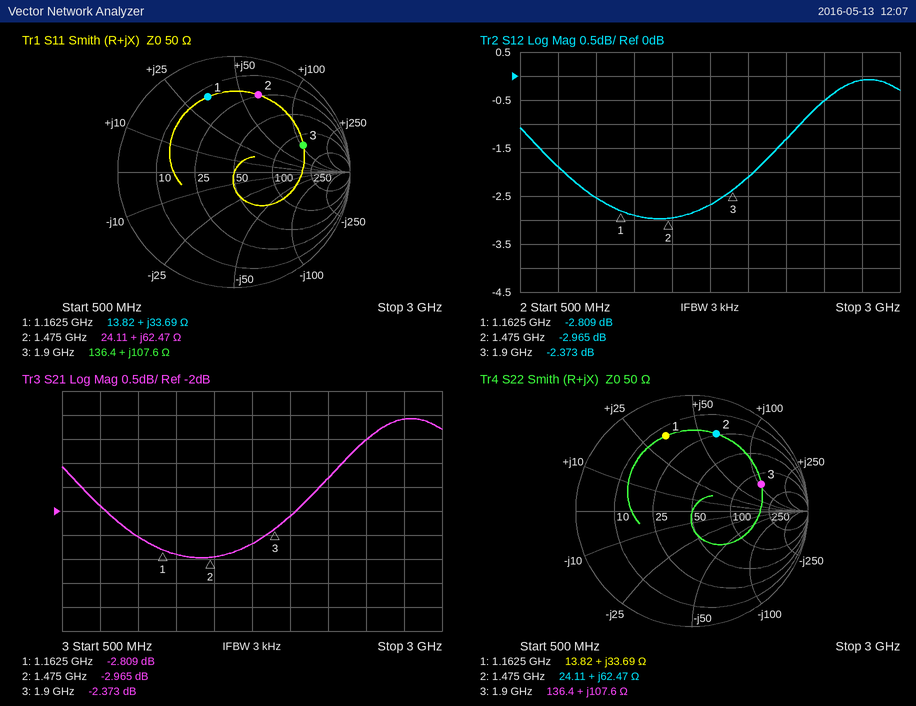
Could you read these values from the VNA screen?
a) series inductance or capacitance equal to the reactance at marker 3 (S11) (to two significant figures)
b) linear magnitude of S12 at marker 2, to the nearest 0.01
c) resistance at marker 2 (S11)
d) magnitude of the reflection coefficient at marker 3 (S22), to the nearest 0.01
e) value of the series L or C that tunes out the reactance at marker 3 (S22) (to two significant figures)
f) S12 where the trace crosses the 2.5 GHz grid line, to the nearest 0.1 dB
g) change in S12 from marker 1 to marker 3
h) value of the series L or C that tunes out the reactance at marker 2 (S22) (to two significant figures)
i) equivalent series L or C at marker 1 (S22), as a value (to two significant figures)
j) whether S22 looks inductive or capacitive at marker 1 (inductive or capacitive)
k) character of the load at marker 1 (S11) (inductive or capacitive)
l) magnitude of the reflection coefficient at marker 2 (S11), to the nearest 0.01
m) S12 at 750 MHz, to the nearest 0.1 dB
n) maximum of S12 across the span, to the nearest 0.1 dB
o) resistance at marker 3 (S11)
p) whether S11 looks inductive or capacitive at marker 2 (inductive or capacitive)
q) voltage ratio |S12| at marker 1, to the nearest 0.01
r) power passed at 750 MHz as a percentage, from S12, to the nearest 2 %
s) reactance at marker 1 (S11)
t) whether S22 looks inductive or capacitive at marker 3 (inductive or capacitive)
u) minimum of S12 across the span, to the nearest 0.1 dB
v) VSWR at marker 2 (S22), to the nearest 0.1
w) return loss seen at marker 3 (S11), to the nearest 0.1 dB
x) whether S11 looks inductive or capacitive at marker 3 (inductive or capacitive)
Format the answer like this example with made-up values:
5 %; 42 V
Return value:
9.0 nH; 0.71; 24.11 Ω; 0.64; 780 fF; -0.5 dB; 0.436 dB; 1.7 pF; 4.6 nH; inductive; inductive; 0.70; -1.9 dB; -0.1 dB; 136.4 Ω; inductive; 0.72; 64 %; +33.69 Ω; inductive; -3.0 dB; 5.6; 3.9 dB; inductive
